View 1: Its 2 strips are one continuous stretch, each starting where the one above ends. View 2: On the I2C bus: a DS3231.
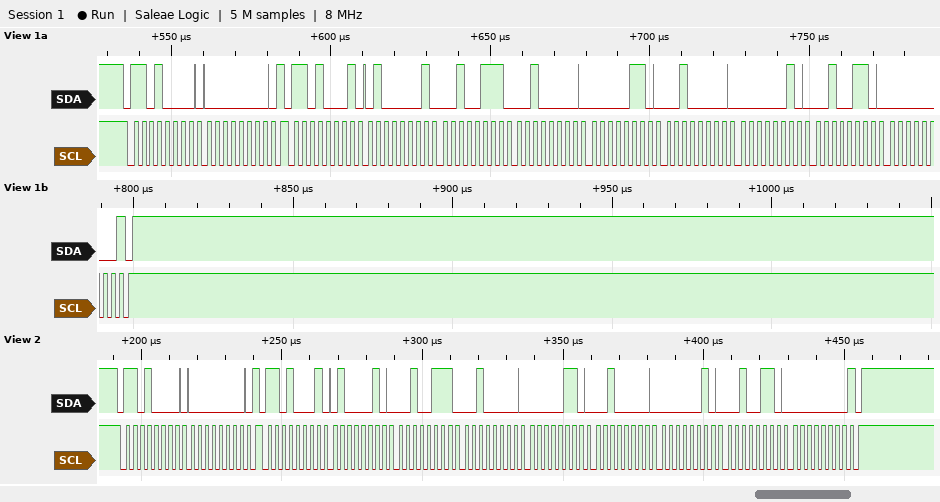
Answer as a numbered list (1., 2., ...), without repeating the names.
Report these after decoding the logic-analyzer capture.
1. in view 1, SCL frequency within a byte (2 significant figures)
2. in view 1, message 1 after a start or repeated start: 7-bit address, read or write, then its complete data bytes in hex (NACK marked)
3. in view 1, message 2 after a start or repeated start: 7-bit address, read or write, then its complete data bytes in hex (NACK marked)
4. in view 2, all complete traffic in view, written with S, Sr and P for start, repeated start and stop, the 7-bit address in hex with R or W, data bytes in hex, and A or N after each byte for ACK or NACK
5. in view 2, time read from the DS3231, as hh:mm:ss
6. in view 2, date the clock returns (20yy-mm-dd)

1. 400 kHz
2. 0x68 write: 00
3. 0x68 read: 41 27 20 06 20 02 26 00 NACK
4. S 68W A 00 A Sr 68R A 42 A 27 A 20 A 06 A 20 A 02 A 26 A 00 N P
5. 20:27:42
6. 2026-02-20
